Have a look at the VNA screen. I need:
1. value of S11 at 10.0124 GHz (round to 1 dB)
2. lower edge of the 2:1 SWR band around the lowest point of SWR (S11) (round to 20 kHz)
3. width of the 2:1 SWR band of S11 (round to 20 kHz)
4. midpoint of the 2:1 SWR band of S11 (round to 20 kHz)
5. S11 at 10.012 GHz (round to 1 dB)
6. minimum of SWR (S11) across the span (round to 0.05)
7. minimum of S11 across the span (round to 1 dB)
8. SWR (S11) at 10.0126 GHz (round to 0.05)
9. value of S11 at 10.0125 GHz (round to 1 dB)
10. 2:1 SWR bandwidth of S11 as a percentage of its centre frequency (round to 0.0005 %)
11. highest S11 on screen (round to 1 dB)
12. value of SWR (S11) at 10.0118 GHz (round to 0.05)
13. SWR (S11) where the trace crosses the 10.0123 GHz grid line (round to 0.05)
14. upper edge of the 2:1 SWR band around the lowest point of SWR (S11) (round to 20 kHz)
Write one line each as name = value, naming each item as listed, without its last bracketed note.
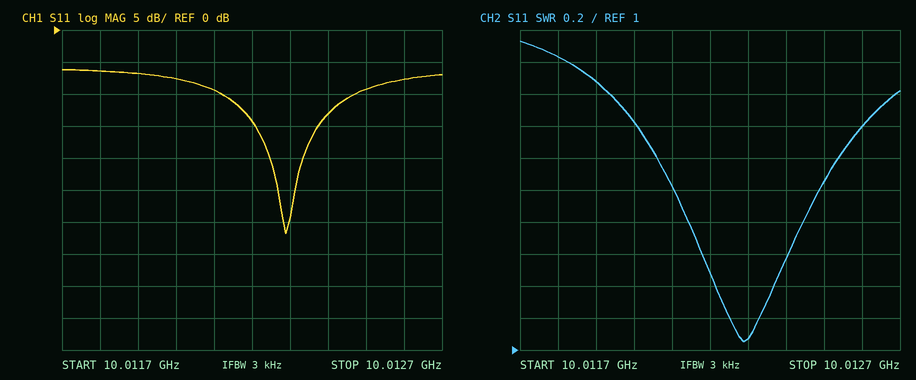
value of S11 at 10.0124 GHz = -13 dB
lower edge of the 2:1 SWR band around the lowest point of SWR (S11) = 10.01210 GHz
width of the 2:1 SWR band of S11 = 380 kHz
midpoint of the 2:1 SWR band of S11 = 10.01230 GHz
S11 at 10.012 GHz = -8 dB
minimum of SWR (S11) across the span = 1.05
minimum of S11 across the span = -32 dB
SWR (S11) at 10.0126 GHz = 2.40
value of S11 at 10.0125 GHz = -9 dB
2:1 SWR bandwidth of S11 as a percentage of its centre frequency = 0.0040 %
highest S11 on screen = -6 dB
value of SWR (S11) at 10.0118 GHz = 2.85
SWR (S11) where the trace crosses the 10.0123 GHz grid line = 1.05
upper edge of the 2:1 SWR band around the lowest point of SWR (S11) = 10.01248 GHz
